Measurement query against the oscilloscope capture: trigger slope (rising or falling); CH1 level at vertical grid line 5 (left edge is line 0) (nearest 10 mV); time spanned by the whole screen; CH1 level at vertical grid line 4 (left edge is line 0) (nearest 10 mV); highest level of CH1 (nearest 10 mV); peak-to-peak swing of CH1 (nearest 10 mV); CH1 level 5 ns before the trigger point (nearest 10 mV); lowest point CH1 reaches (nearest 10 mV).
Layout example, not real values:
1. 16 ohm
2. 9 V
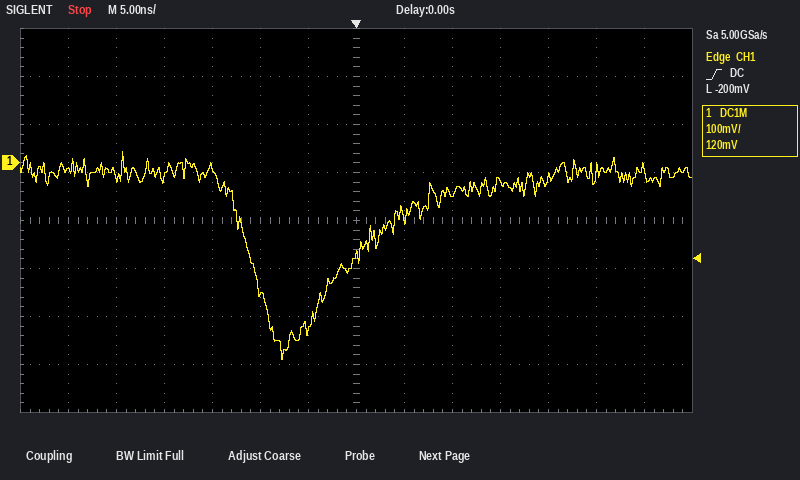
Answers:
1. rising
2. -270 mV
3. 70 ns
4. -10 mV
5. 20 mV
6. 430 mV
7. -350 mV
8. -410 mV
